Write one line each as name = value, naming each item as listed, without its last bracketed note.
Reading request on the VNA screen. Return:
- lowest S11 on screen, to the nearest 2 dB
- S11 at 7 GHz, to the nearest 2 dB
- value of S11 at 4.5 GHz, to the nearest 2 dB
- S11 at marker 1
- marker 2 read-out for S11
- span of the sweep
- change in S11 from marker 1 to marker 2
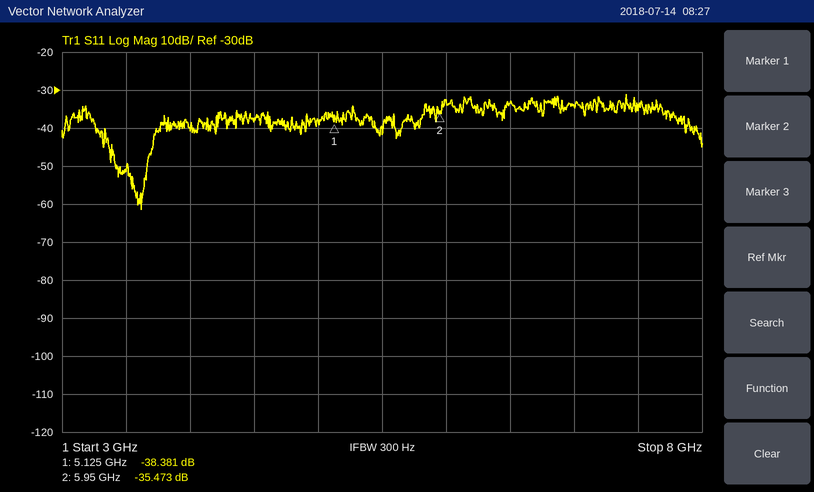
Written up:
lowest S11 on screen, to the nearest 2 dB = -62 dB
S11 at 7 GHz, to the nearest 2 dB = -34 dB
value of S11 at 4.5 GHz, to the nearest 2 dB = -38 dB
S11 at marker 1 = -38.381 dB
marker 2 read-out for S11 = -35.473 dB
span of the sweep = 5 GHz
change in S11 from marker 1 to marker 2 = 2.908 dB
